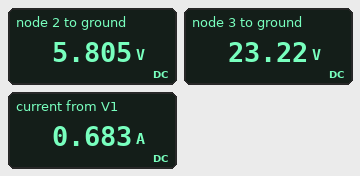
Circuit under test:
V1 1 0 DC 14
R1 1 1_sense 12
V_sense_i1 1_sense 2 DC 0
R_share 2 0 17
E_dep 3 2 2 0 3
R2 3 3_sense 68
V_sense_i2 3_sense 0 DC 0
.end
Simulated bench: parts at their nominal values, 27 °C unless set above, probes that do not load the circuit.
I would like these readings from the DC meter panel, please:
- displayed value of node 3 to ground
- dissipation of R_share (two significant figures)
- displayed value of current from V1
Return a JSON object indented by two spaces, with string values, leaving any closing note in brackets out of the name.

{
  "displayed value of node 3 to ground": "23.22 V",
  "dissipation of R_share": "2.0 W",
  "displayed value of current from V1": "0.683 A"
}
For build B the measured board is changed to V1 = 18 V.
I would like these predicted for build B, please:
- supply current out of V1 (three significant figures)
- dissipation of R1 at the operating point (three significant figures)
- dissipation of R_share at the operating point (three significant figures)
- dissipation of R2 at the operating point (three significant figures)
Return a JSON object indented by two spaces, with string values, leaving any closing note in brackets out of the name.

{
  "supply current out of V1": "878 mA",
  "dissipation of R1 at the operating point": "9.25 W",
  "dissipation of R_share at the operating point": "3.28 W",
  "dissipation of R2 at the operating point": "13.1 W"
}
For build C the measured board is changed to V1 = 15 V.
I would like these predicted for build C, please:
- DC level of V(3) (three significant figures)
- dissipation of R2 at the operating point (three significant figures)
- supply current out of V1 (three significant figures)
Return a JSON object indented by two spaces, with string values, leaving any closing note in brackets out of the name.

{
  "DC level of V(3)": "24.9 V",
  "dissipation of R2 at the operating point": "9.10 W",
  "supply current out of V1": "732 mA"
}
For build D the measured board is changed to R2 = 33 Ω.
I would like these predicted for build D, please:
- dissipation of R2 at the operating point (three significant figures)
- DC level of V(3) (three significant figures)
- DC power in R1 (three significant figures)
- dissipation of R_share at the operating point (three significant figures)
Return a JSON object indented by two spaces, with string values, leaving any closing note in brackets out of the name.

{
  "dissipation of R2 at the operating point": "9.51 W",
  "DC level of V(3)": "17.7 V",
  "DC power in R1": "7.63 W",
  "dissipation of R_share at the operating point": "1.15 W"
}
